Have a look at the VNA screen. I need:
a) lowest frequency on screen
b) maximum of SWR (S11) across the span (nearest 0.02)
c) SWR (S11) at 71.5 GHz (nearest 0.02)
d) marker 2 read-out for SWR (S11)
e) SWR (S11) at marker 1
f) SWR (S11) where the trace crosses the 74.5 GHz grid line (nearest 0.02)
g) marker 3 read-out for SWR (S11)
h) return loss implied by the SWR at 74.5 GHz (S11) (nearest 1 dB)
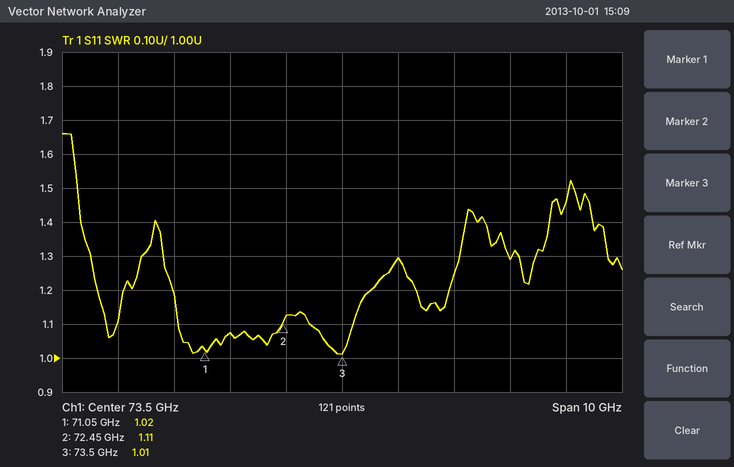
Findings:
68.5 GHz
1.66
1.08
1.11
1.02
1.30
1.01
18 dB
